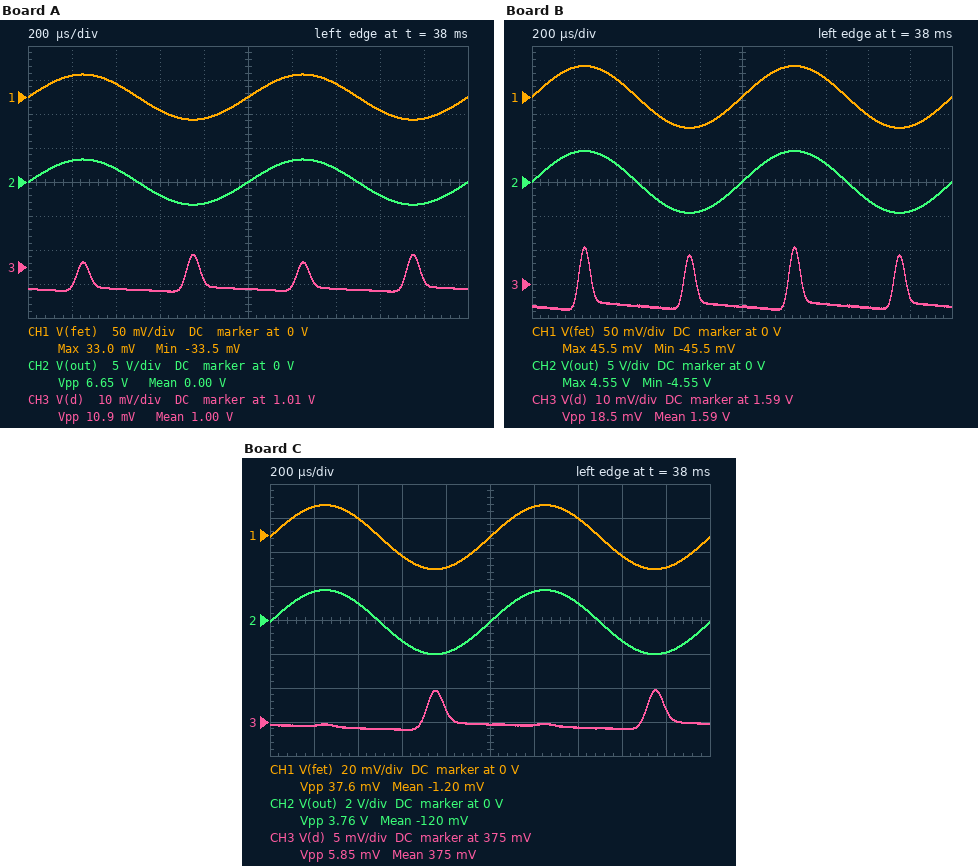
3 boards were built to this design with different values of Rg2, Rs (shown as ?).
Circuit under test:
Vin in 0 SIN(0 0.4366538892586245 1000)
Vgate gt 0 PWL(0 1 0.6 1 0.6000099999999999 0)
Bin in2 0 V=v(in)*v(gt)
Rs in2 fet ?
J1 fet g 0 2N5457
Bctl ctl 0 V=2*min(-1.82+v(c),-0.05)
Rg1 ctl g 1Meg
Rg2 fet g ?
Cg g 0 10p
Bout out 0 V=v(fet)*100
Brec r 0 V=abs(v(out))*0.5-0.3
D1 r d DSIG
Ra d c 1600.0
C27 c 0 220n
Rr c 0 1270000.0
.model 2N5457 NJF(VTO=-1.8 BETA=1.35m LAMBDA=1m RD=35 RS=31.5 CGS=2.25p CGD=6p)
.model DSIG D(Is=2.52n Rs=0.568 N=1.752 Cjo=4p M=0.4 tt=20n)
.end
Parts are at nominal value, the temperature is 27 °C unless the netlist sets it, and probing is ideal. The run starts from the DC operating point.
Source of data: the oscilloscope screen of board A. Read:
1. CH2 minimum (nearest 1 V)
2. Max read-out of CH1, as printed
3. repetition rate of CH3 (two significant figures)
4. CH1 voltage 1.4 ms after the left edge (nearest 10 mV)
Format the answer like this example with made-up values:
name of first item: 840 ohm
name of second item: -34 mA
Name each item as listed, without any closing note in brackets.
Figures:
CH2 minimum: -3 V
Max read-out of CH1, as printed: 33.0 mV
repetition rate of CH3: 2.0 kHz
CH1 voltage 1.4 ms after the left edge: 20 mV
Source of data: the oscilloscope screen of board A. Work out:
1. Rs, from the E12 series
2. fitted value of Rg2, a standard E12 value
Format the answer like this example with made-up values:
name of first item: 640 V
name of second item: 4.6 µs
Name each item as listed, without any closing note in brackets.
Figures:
Rs, from the E12 series: 6.8 kΩ
fitted value of Rg2, a standard E12 value: 1.8 MΩ
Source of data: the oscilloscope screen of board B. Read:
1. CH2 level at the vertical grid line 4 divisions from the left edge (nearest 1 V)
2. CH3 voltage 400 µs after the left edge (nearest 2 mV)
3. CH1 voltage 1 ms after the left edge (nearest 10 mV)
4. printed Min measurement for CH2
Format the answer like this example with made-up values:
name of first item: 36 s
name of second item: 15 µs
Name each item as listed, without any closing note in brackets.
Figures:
CH2 level at the vertical grid line 4 divisions from the left edge: -4 V
CH3 voltage 400 µs after the left edge: 1.584 V
CH1 voltage 1 ms after the left edge: 0 V
printed Min measurement for CH2: -4.55 V
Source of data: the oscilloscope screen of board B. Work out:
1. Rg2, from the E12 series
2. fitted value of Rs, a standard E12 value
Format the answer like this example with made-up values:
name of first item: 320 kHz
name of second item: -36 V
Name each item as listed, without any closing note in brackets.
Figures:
Rg2, from the E12 series: 1.8 MΩ
fitted value of Rs, a standard E12 value: 2.7 kΩ
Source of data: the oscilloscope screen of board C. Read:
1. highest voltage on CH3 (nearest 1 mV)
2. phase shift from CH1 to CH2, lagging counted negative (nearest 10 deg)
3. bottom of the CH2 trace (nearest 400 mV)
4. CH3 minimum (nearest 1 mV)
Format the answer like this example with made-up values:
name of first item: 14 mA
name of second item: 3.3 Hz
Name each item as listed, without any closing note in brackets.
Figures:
highest voltage on CH3: 380 mV
phase shift from CH1 to CH2, lagging counted negative: 0 deg
bottom of the CH2 trace: -2.0 V
CH3 minimum: 374 mV
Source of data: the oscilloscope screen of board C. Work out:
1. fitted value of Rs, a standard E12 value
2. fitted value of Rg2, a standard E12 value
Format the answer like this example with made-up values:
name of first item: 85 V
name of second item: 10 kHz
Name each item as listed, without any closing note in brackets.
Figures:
fitted value of Rs, a standard E12 value: 18 kΩ
fitted value of Rg2, a standard E12 value: 820 kΩ
